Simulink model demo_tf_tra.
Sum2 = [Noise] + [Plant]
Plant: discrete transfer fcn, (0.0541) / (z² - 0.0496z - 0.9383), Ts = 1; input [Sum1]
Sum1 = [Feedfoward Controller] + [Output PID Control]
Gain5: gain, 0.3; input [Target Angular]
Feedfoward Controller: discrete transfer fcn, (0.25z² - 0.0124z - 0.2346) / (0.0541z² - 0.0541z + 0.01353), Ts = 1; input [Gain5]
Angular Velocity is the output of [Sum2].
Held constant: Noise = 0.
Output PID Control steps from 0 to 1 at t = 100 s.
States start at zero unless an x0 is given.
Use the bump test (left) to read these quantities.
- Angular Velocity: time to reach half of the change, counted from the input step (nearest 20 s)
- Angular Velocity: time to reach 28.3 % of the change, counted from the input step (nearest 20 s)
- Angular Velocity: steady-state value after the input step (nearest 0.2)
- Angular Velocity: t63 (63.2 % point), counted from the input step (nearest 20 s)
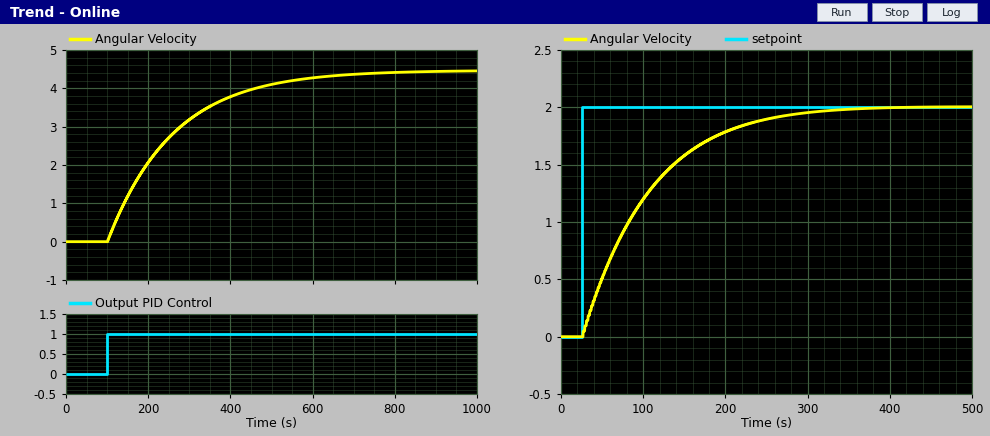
120 s
60 s
4.4
160 s
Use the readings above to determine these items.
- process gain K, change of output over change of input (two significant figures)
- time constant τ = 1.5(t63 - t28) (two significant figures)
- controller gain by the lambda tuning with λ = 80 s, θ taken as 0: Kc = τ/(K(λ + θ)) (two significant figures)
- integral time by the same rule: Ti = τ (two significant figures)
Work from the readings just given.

4.4
150 s
0.43
150 s
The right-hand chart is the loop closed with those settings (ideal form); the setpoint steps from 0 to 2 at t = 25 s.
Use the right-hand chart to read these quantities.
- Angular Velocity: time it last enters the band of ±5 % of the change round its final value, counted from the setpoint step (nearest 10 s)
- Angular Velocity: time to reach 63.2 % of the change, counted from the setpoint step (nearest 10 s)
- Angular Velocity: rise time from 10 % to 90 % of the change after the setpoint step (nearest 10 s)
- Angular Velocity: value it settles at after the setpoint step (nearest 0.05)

230 s
80 s
170 s
2.00
